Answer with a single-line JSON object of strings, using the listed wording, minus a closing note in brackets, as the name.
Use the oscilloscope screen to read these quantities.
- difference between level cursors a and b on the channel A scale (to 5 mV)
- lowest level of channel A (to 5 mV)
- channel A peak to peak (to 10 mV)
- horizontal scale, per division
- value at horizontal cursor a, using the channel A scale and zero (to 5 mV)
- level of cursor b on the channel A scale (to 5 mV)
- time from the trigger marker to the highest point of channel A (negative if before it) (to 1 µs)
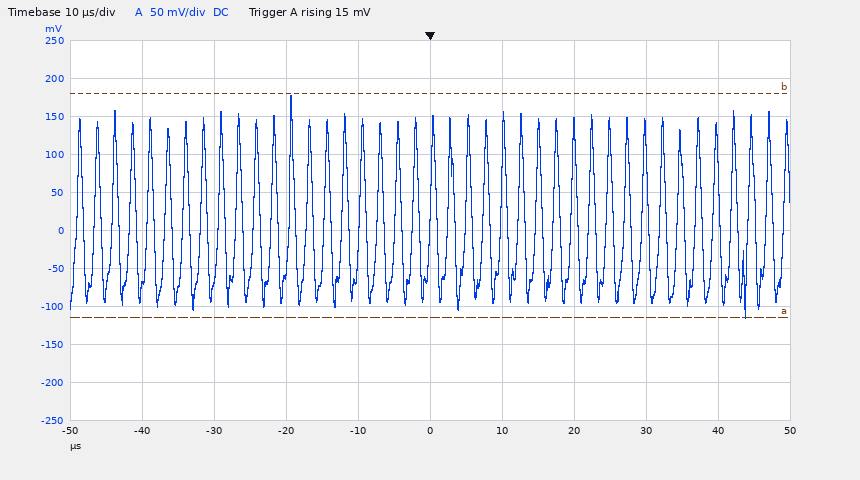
{"difference between level cursors a and b on the channel A scale": "295 mV", "lowest level of channel A": "-115 mV", "channel A peak to peak": "290 mV", "horizontal scale, per division": "10 µs", "value at horizontal cursor a, using the channel A scale and zero": "-115 mV", "level of cursor b on the channel A scale": "180 mV", "time from the trigger marker to the highest point of channel A (negative if before it)": "-19 µs"}
